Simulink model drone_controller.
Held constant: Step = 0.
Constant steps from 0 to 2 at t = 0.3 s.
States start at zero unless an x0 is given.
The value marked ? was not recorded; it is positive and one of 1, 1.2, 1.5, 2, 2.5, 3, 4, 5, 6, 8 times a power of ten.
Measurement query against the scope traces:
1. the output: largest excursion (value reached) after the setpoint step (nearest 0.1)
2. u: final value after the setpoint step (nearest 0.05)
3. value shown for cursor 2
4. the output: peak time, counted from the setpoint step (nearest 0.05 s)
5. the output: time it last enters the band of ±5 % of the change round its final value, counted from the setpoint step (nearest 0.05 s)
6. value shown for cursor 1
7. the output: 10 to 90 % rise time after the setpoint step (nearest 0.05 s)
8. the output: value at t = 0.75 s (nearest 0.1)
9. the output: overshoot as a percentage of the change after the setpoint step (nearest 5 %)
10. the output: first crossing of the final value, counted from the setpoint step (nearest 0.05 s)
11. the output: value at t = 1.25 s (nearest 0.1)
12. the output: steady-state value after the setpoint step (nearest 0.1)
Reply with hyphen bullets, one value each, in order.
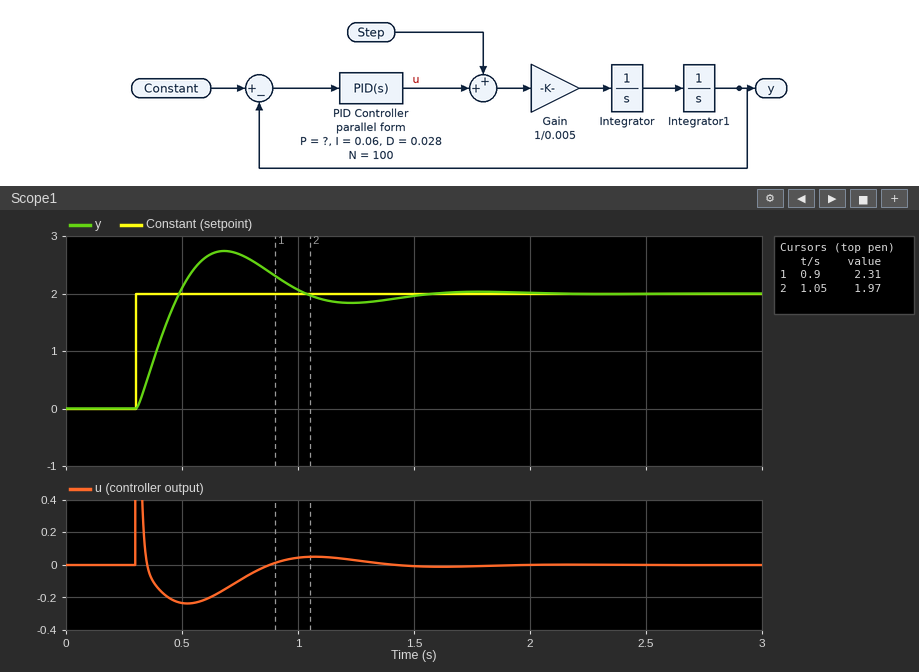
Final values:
- 2.7
- 0.00
- 1.97
- 0.40 s
- 1.10 s
- 2.31
- 0.15 s
- 2.7
- 35 %
- 0.20 s
- 1.8
- 2.0
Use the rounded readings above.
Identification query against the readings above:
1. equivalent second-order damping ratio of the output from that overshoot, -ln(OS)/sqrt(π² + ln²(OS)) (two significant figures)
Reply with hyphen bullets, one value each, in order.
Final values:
- 0.32
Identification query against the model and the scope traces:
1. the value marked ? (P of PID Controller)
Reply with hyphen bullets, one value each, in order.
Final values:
- 0.2
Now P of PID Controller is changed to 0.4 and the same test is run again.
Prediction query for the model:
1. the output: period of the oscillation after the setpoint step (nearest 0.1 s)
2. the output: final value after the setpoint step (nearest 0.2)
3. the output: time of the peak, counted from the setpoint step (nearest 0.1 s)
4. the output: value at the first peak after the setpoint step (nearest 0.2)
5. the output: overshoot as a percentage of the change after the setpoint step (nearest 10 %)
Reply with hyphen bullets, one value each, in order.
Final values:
- 0.7 s
- 2.0
- 0.3 s
- 3.0
- 50 %
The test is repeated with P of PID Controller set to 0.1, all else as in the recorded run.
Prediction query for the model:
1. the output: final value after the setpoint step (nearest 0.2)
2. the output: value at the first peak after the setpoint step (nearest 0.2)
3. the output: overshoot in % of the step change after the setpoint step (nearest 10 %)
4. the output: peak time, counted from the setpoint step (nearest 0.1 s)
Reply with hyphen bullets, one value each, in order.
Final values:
- 2.0
- 2.6
- 30 %
- 0.5 s
